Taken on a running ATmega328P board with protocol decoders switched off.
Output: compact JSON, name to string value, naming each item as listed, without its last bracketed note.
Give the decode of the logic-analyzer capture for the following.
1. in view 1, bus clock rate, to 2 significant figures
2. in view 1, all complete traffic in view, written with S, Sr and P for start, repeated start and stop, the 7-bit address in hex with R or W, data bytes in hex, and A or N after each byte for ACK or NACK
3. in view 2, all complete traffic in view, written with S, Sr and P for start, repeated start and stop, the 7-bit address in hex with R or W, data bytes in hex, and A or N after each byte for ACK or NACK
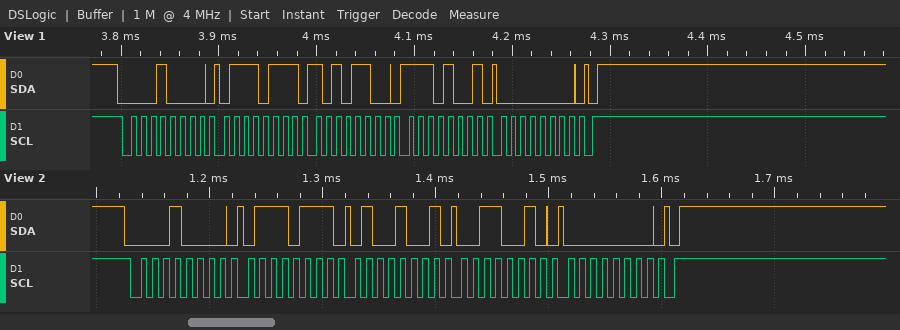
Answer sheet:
{"in view 1, bus clock rate, to 2 significant figures": "100 kHz", "in view 1, all complete traffic in view, written with S, Sr and P for start, repeated start and stop, the 7-bit address in hex with R or W, data bytes in hex, and A or N after each byte for ACK or NACK": "S 08W A 77 A AC A E9 A 00 A P", "in view 2, all complete traffic in view, written with S, Sr and P for start, repeated start and stop, the 7-bit address in hex with R or W, data bytes in hex, and A or N after each byte for ACK or NACK": "S 08W A 77 A 49 A 32 A 00 A P"}
